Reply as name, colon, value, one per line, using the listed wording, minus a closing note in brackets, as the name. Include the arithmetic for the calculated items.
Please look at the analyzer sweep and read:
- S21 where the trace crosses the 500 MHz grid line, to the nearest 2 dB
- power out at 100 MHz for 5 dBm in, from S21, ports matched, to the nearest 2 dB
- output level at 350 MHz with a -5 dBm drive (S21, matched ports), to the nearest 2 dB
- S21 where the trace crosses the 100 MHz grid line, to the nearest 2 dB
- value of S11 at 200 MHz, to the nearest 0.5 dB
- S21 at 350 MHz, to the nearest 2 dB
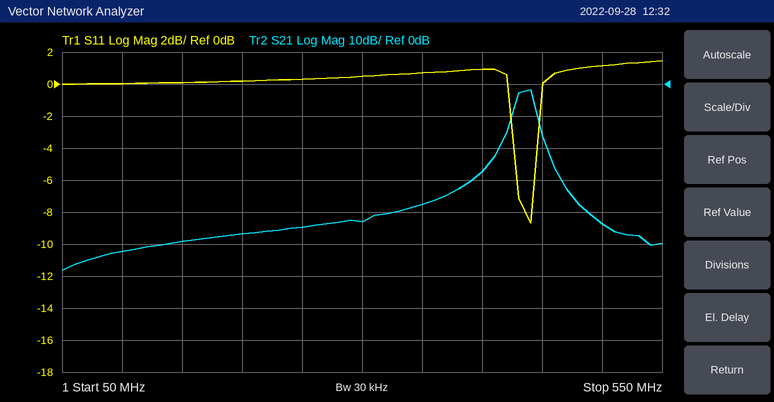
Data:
S21 where the trace crosses the 500 MHz grid line, to the nearest 2 dB: -44 dB
power out at 100 MHz for 5 dBm in, from S21, ports matched, to the nearest 2 dB: 5 dBm + (-52 dB) = -48 dBm
output level at 350 MHz with a -5 dBm drive (S21, matched ports), to the nearest 2 dB: -5 dBm + (-38 dB) = -42 dBm
S21 where the trace crosses the 100 MHz grid line, to the nearest 2 dB: -52 dB
value of S11 at 200 MHz, to the nearest 0.5 dB: 0.0 dB
S21 at 350 MHz, to the nearest 2 dB: -38 dB
